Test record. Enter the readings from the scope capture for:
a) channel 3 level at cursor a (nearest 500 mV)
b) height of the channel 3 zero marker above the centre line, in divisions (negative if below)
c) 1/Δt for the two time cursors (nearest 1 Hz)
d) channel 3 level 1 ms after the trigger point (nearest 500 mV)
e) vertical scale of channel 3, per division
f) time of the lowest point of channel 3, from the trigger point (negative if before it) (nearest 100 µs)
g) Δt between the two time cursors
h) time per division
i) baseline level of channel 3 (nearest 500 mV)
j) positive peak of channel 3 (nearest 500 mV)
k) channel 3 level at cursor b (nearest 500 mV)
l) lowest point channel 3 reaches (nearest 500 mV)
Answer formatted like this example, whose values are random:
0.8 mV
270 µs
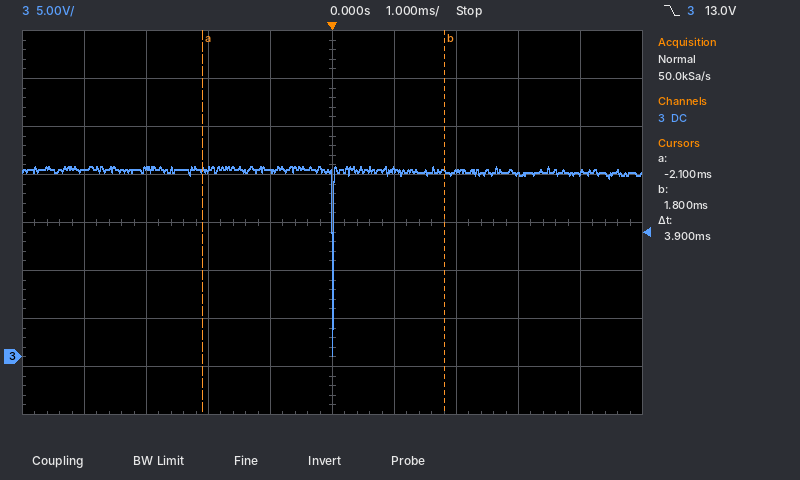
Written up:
19.5 V
-2.8 div
256 Hz
19.5 V
5 V
0.0 ms
3.9 ms
1 ms
19.5 V
20.0 V
19.5 V
0.0 V
